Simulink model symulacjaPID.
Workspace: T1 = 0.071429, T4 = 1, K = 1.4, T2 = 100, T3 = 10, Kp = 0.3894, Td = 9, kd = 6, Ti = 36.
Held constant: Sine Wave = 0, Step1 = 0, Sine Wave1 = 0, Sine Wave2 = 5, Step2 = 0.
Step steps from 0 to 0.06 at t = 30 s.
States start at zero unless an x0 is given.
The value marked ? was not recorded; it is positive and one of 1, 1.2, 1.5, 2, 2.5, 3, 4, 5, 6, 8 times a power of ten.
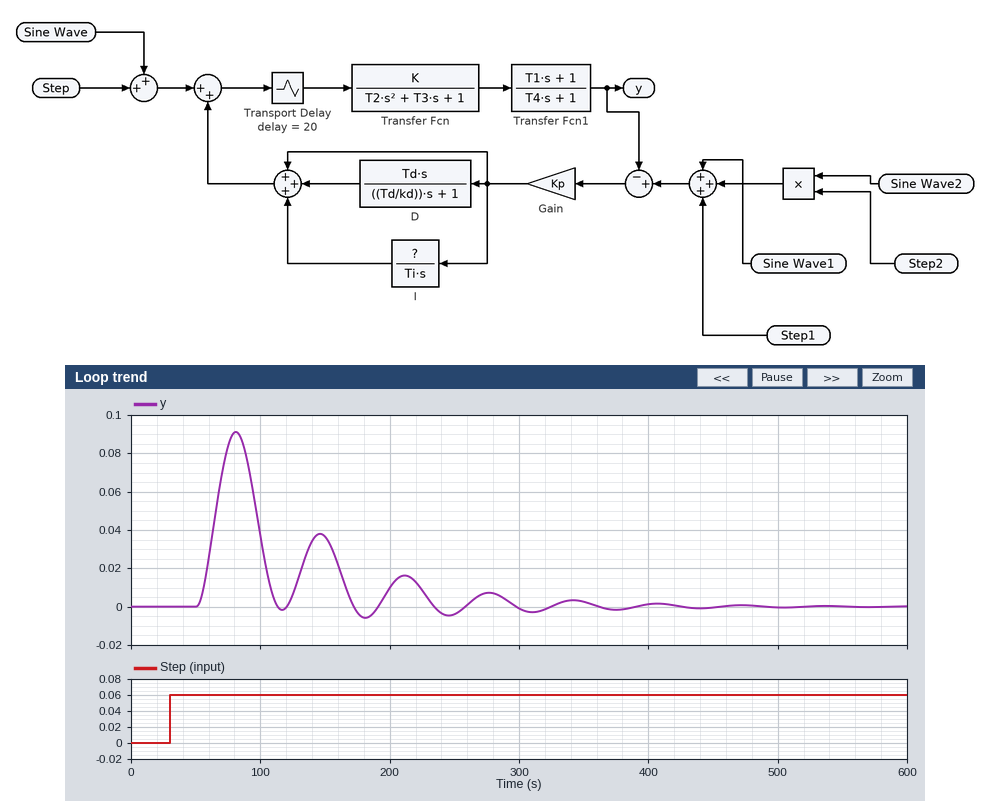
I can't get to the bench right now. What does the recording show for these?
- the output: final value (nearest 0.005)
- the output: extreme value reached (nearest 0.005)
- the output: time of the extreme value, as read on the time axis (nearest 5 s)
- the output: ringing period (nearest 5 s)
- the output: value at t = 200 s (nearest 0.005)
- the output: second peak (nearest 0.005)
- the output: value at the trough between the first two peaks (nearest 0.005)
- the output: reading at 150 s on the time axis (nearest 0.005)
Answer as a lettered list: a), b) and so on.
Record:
a) 0.000
b) 0.090
c) 80 s
d) 65 s
e) 0.010
f) 0.040
g) 0.000
h) 0.035
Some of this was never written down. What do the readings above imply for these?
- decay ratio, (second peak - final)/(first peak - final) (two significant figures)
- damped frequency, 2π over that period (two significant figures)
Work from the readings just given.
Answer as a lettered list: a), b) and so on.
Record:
a) 0.44
b) 0.097 rad/s
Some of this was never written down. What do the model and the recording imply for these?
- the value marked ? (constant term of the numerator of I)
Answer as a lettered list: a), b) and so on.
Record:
a) 1.2
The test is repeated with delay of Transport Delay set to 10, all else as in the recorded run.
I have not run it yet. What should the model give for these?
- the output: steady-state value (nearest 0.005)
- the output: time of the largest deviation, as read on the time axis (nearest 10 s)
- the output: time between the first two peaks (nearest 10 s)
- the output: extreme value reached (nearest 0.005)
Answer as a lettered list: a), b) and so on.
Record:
a) 0.000
b) 70 s
c) 50 s
d) 0.075
